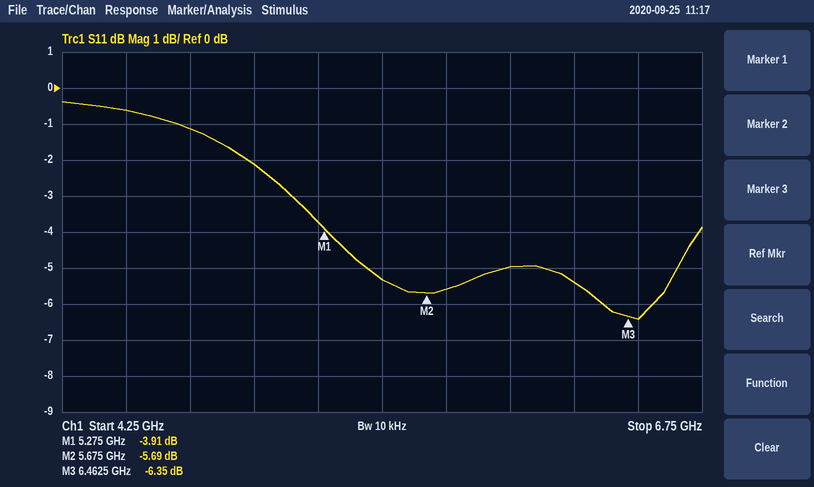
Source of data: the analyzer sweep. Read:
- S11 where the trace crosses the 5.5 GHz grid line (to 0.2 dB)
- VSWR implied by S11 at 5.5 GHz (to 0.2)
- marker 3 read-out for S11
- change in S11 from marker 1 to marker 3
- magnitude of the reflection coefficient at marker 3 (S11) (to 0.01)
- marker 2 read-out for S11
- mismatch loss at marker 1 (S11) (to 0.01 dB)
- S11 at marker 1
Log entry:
-5.4 dB
3.4
-6.35 dB
-2.44 dB
0.48
-5.69 dB
2.27 dB
-3.91 dB
